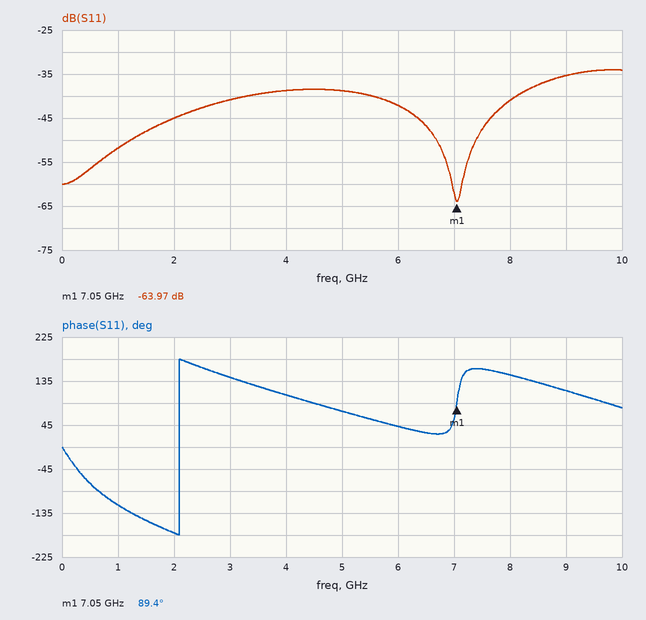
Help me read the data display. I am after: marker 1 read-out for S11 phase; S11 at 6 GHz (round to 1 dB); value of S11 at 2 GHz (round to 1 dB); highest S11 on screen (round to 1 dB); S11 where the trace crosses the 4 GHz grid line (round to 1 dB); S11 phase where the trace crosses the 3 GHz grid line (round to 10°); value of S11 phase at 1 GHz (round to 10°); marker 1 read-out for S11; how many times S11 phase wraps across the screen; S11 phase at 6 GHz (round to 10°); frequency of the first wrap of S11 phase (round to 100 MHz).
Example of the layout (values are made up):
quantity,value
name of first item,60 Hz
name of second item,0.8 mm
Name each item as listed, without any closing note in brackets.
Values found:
quantity,value
marker 1 read-out for S11 phase,89.4°
S11 at 6 GHz,-42 dB
value of S11 at 2 GHz,-45 dB
highest S11 on screen,-34 dB
S11 where the trace crosses the 4 GHz grid line,-39 dB
S11 phase where the trace crosses the 3 GHz grid line,140°
value of S11 phase at 1 GHz,-120°
marker 1 read-out for S11,-63.97 dB
how many times S11 phase wraps across the screen,1
S11 phase at 6 GHz,40°
frequency of the first wrap of S11 phase,2.1 GHz
